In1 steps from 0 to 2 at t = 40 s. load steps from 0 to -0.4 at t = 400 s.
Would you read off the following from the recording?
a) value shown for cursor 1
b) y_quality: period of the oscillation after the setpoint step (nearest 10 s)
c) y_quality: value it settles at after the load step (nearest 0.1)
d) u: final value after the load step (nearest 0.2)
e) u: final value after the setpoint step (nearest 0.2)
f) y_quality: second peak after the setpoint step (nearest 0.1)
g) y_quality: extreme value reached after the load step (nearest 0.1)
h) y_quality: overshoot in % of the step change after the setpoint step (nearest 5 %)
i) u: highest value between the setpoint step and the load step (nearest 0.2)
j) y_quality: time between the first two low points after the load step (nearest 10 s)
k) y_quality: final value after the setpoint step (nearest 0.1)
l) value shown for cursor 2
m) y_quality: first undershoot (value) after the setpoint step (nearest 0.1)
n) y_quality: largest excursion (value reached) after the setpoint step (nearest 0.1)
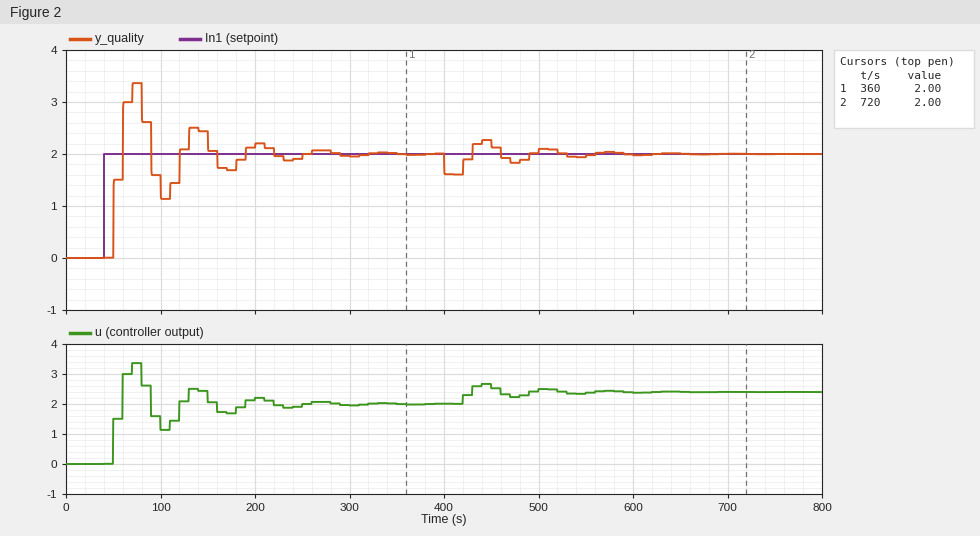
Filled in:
2.00
60 s
2.0
2.4
2.0
2.5
1.6
70 %
3.4
60 s
2.0
2.00
1.1
3.4
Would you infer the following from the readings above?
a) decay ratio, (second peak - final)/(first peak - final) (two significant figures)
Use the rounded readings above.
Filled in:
0.36
